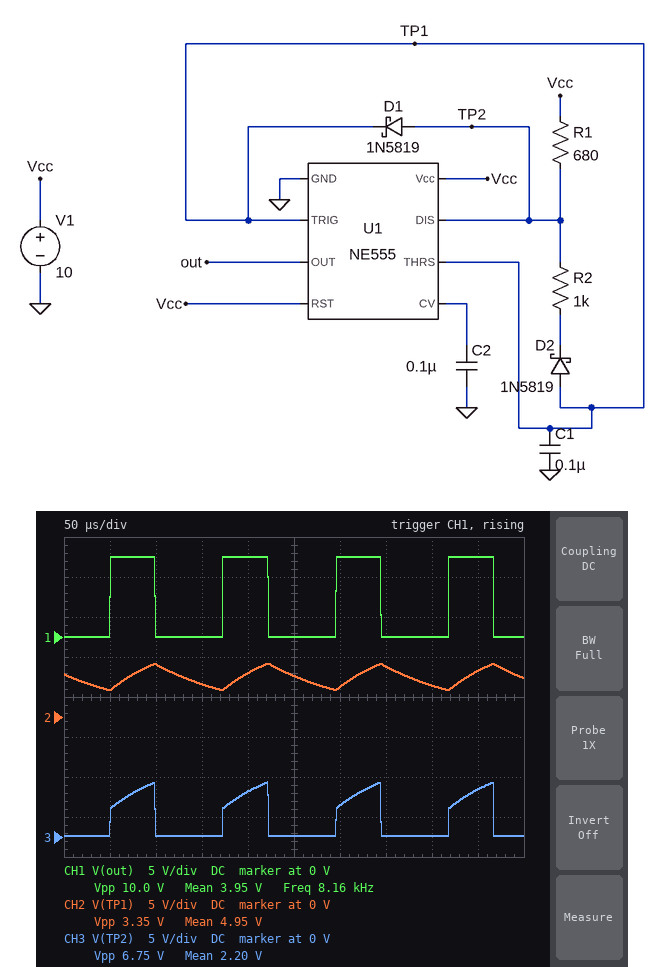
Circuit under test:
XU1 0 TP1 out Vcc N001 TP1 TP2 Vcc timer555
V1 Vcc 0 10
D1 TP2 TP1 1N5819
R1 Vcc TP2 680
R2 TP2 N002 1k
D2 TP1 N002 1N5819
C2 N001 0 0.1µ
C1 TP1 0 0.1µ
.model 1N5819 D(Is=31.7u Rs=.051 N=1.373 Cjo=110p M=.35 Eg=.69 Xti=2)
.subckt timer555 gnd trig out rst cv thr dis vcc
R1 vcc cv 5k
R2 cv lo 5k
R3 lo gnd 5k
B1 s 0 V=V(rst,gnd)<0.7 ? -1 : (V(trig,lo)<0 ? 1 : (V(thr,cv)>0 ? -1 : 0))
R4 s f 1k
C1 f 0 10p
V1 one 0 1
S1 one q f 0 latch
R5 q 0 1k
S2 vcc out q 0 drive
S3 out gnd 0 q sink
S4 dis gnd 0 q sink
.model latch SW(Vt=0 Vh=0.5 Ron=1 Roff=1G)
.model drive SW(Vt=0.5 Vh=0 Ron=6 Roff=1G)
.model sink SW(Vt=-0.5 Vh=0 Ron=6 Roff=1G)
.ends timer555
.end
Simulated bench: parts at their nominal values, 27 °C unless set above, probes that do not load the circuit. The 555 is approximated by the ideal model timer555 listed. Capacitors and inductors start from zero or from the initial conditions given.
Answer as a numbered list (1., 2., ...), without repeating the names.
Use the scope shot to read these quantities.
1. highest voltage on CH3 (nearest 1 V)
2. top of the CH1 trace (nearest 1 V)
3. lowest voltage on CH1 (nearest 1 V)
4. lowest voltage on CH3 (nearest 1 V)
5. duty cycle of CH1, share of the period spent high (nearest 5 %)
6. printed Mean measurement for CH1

1. 7 V
2. 10 V
3. 0 V
4. 0 V
5. 40 %
6. 3.95 V
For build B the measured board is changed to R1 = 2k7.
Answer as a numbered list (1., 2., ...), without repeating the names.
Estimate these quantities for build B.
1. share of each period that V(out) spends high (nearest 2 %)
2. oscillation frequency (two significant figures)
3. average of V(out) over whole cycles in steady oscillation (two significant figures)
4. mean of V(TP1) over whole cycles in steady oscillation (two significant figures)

1. 72 %
2. 3.8 kHz
3. 7.3 V
4. 5.1 V
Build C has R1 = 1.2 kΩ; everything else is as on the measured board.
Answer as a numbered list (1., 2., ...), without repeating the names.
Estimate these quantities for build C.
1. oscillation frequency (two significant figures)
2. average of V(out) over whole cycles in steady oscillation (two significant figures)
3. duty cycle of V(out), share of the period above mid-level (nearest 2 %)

1. 6.3 kHz
2. 5.4 V
3. 54 %
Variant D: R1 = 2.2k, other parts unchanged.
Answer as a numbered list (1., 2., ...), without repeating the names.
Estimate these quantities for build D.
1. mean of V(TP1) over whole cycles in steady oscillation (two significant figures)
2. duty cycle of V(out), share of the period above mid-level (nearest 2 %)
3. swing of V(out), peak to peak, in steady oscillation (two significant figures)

1. 5.1 V
2. 68 %
3. 10 V
